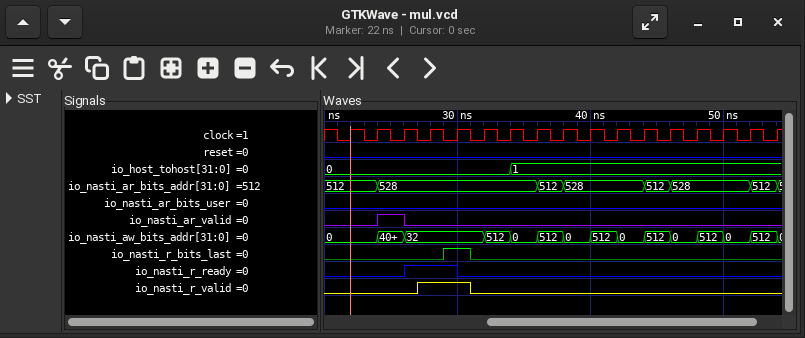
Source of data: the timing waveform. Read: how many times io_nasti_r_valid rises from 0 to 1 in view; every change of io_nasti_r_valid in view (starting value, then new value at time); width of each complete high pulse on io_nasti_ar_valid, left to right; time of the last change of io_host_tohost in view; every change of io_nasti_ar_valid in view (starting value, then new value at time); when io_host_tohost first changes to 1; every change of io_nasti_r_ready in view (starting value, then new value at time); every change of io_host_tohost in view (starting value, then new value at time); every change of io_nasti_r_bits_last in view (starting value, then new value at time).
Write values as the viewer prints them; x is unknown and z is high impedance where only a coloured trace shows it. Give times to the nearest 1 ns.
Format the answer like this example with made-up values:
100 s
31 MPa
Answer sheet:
1
0, 1 at 27 ns, 0 at 31 ns
2 ns
34 ns
0, 1 at 24 ns, 0 at 26 ns
34 ns
0, 1 at 26 ns, 0 at 30 ns
0, 1 at 34 ns
0, 1 at 29 ns, 0 at 31 ns
